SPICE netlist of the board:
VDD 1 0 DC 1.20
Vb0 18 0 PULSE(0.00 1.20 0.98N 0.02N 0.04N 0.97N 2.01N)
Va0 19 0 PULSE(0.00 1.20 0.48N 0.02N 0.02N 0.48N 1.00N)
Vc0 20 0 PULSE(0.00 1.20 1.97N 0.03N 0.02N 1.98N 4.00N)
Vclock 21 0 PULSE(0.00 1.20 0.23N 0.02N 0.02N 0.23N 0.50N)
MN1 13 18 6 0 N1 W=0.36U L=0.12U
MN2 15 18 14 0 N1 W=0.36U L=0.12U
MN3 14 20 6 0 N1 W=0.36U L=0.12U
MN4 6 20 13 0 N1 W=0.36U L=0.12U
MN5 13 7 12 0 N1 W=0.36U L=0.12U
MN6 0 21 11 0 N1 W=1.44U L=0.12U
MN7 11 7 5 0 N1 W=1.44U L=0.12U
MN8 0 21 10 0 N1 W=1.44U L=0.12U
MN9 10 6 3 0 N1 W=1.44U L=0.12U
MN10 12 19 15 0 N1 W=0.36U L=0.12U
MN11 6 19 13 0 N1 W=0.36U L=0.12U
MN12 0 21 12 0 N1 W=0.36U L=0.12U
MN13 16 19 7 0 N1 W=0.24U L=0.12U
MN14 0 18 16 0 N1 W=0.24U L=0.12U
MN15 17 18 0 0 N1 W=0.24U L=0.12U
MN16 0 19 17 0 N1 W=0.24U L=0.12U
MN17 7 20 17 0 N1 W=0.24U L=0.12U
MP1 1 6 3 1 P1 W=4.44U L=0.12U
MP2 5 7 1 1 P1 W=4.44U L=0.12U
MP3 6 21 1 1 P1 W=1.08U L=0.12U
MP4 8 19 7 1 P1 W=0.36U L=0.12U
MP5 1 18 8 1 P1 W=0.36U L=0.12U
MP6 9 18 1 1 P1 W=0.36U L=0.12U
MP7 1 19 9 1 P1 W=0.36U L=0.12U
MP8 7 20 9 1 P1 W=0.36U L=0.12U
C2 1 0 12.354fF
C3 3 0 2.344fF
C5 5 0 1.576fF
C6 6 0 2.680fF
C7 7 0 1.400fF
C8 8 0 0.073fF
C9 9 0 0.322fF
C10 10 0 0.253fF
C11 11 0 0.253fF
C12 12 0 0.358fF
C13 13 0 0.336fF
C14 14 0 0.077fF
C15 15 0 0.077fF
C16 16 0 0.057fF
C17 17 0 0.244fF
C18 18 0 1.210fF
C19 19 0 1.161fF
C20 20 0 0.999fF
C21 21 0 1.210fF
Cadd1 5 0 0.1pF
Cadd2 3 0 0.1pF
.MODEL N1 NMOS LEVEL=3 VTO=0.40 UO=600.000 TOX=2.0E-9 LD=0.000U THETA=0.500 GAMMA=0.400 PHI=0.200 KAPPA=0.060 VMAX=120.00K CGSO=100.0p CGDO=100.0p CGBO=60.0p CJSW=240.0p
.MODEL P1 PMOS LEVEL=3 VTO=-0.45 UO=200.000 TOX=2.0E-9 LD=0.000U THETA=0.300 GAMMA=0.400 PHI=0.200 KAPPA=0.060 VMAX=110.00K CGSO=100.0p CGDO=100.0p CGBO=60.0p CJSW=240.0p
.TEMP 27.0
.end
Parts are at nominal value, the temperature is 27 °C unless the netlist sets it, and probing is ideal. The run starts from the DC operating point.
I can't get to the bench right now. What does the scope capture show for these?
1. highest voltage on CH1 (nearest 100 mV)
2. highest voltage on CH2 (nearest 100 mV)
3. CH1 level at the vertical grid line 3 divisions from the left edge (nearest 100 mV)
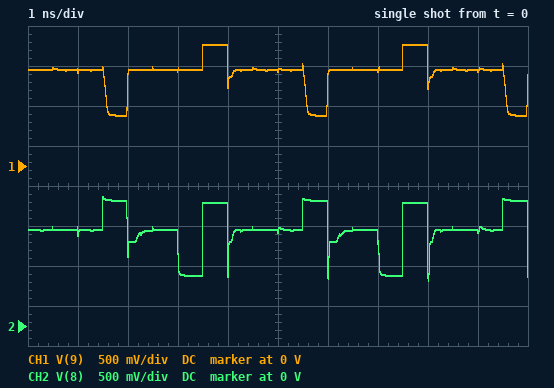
1.5 V
1.6 V
1.2 V
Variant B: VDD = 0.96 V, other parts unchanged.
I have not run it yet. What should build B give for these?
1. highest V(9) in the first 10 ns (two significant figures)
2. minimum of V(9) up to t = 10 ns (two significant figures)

1.4 V
580 mV
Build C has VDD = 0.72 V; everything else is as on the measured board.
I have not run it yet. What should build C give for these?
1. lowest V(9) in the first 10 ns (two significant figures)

530 mV
